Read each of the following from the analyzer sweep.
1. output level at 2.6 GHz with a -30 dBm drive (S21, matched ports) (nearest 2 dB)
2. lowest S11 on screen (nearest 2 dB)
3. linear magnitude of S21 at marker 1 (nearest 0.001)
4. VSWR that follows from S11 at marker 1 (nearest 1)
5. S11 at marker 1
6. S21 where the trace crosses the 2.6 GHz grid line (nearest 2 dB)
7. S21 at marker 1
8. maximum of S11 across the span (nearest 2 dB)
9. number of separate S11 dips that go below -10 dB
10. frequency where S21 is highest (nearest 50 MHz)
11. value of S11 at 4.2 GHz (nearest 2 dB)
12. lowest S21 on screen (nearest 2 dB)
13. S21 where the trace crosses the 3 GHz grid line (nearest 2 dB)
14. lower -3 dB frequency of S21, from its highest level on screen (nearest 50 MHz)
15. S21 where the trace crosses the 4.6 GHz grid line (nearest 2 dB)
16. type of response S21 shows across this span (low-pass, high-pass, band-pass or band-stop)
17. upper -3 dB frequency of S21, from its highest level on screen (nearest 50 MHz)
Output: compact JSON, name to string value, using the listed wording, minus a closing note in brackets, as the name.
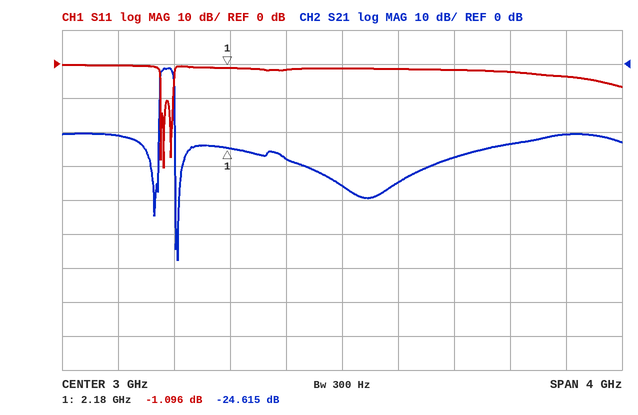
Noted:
{"output level at 2.6 GHz with a -30 dBm drive (S21, matched ports)": "-58 dBm", "lowest S11 on screen": "-30 dB", "linear magnitude of S21 at marker 1": "0.059", "VSWR that follows from S11 at marker 1": "16", "S11 at marker 1": "-1.096 dB", "S21 where the trace crosses the 2.6 GHz grid line": "-28 dB", "S21 at marker 1": "-24.615 dB", "maximum of S11 across the span": "0 dB", "number of separate S11 dips that go below -10 dB": "3", "frequency where S21 is highest": "1.75 GHz", "value of S11 at 4.2 GHz": "-2 dB", "lowest S21 on screen": "-58 dB", "S21 where the trace crosses the 3 GHz grid line": "-36 dB", "lower -3 dB frequency of S21, from its highest level on screen": "1.70 GHz", "S21 where the trace crosses the 4.6 GHz grid line": "-20 dB", "type of response S21 shows across this span": "band-pass", "upper -3 dB frequency of S21, from its highest level on screen": "1.80 GHz"}
